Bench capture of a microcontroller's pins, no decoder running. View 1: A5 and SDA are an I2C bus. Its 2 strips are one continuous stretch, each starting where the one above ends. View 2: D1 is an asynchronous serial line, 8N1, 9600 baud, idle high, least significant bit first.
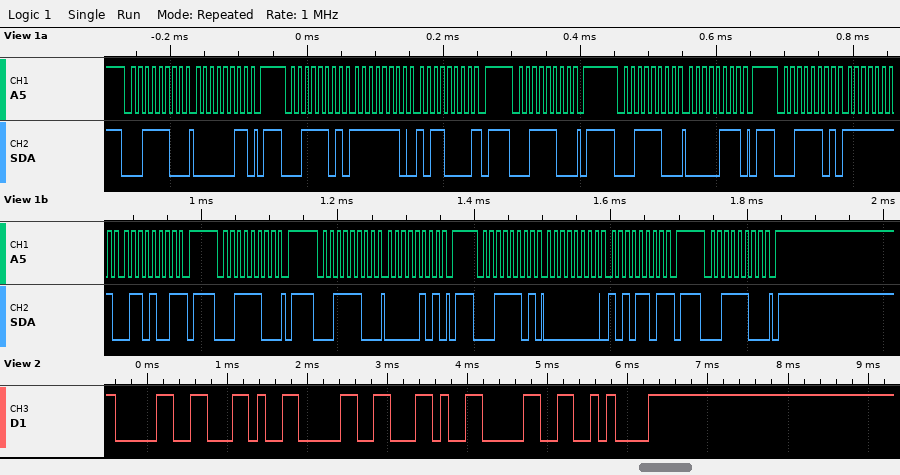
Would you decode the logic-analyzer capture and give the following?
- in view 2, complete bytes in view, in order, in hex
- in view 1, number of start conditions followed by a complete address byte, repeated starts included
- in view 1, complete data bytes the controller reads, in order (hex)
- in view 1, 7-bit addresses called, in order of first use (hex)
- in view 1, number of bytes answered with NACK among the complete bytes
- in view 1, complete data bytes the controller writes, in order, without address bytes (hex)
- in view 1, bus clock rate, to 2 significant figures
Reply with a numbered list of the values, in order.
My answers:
1. 30 2C 30 2C 30 0A
2. 9
3. FE B0 FF 69 00 AD
4. 0x1E
5. 3
6. 03 07 05
7. 100 kHz
